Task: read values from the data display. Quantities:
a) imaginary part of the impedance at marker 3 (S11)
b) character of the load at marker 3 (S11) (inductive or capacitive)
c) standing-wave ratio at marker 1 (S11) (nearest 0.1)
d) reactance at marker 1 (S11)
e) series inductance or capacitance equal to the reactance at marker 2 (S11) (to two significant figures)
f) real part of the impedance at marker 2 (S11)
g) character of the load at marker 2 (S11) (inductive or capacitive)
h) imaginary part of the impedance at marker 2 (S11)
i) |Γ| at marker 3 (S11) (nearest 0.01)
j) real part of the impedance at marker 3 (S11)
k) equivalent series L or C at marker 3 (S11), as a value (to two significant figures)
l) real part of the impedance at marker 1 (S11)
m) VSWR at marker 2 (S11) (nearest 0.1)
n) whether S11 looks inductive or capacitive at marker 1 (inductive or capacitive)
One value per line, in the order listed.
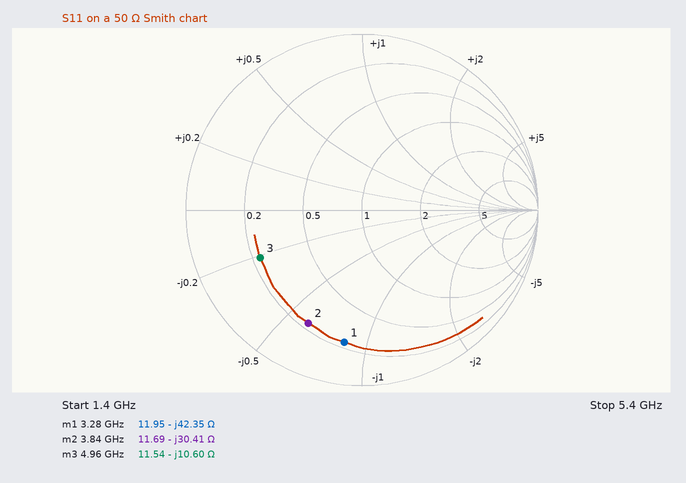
-10.60 Ω
capacitive
7.3
-42.35 Ω
1.4 pF
11.69 Ω
capacitive
-30.41 Ω
0.64
11.54 Ω
3.0 pF
11.95 Ω
5.9
capacitive
